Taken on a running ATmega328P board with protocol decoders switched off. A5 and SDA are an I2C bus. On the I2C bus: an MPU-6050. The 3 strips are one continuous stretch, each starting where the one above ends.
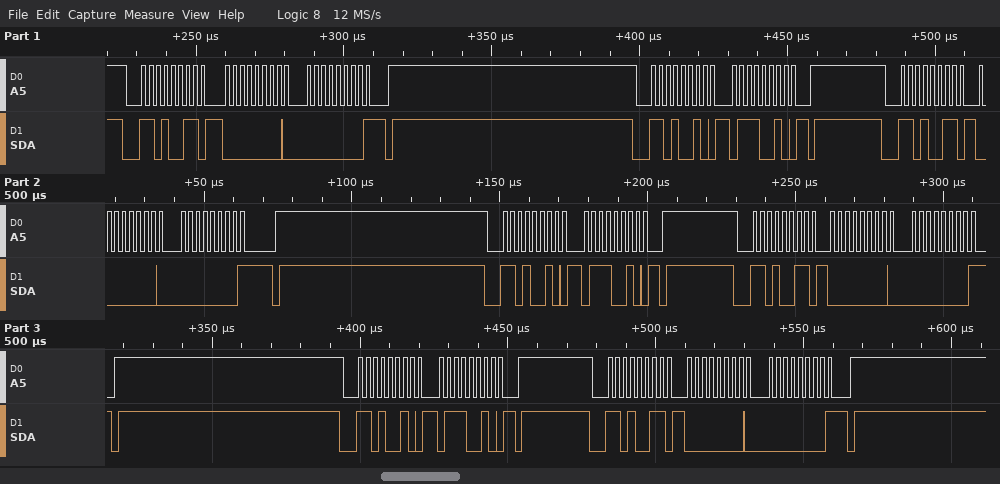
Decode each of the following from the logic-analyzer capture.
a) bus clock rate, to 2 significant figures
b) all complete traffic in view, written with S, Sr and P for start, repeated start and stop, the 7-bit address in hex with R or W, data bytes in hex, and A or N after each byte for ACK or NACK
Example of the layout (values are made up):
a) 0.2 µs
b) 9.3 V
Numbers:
a) 400 kHz
b) S 69R A 00 A 00 N P S 69W A 72 A P S 69R A 00 A 00 N P S 69W A 72 A P S 69R A 00 A 00 N P S 69W A 72 A P S 69R A 00 A 00 N P
